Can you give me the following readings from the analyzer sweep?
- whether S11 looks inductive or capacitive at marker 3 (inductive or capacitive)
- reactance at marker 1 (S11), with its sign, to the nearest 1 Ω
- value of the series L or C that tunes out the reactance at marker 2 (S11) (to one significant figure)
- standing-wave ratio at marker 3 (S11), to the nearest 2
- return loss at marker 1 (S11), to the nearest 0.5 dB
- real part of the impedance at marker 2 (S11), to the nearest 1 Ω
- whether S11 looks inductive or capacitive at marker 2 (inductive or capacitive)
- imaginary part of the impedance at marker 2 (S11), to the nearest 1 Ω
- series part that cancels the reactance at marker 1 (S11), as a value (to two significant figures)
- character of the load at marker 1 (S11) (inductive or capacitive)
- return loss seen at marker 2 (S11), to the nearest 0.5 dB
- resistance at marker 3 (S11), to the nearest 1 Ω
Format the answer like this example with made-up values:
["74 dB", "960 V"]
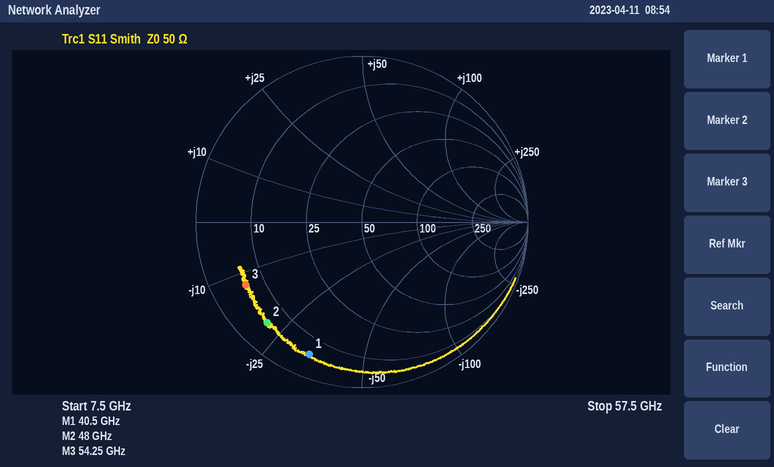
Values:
["capacitive", "-34 Ω", "70 pH", "8", "1.5 dB", "5 Ω", "capacitive", "-21 Ω", "130 pH", "capacitive", "1.5 dB", "6 Ω"]
